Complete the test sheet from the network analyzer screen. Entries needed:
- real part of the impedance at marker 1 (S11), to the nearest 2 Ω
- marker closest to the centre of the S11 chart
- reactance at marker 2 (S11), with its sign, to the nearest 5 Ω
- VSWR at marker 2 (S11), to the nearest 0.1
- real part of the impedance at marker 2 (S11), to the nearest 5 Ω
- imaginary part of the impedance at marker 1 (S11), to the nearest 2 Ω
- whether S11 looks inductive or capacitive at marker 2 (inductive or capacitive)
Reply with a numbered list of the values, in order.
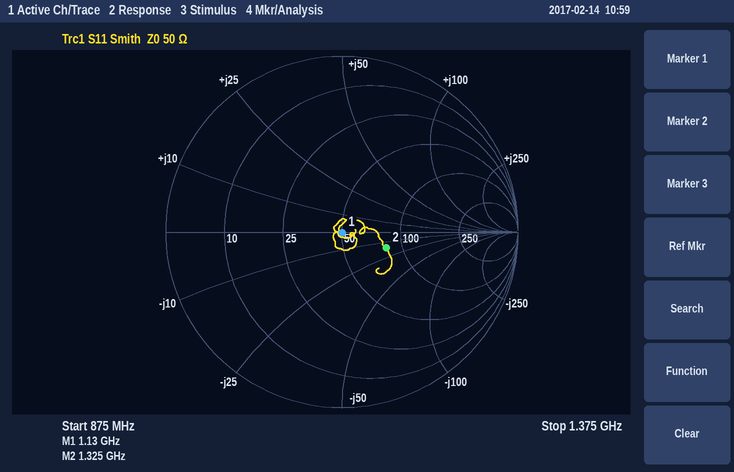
1. 50 Ω
2. marker 1
3. -15 Ω
4. 1.7
5. 80 Ω
6. 0 Ω
7. capacitive
